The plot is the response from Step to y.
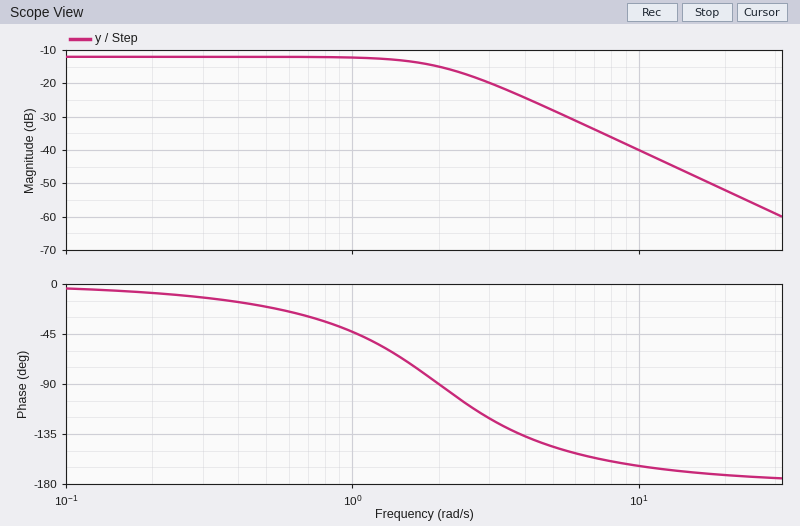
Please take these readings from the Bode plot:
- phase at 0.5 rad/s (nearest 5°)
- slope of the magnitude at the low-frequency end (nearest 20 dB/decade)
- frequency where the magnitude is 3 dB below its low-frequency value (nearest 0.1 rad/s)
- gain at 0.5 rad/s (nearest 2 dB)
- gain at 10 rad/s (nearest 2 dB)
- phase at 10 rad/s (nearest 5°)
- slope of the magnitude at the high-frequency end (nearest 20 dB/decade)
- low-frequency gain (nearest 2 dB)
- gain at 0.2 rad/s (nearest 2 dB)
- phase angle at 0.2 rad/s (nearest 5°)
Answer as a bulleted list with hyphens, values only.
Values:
- -20°
- 0 dB/decade
- 2.0 rad/s
- -12 dB
- -40 dB
- -165°
- -40 dB/decade
- -12 dB
- -12 dB
- -10°
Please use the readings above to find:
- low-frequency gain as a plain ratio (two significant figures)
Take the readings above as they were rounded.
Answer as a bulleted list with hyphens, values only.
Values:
- 0.25
